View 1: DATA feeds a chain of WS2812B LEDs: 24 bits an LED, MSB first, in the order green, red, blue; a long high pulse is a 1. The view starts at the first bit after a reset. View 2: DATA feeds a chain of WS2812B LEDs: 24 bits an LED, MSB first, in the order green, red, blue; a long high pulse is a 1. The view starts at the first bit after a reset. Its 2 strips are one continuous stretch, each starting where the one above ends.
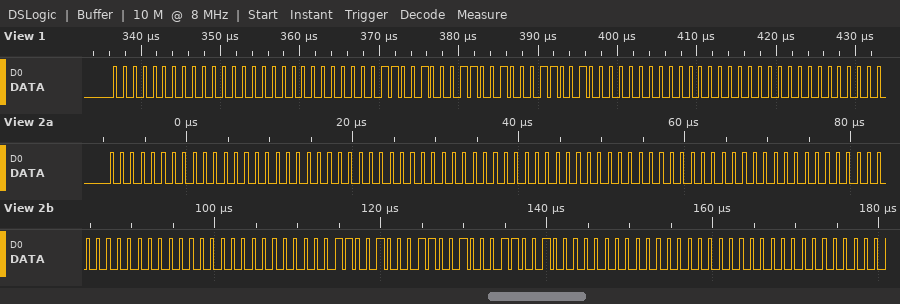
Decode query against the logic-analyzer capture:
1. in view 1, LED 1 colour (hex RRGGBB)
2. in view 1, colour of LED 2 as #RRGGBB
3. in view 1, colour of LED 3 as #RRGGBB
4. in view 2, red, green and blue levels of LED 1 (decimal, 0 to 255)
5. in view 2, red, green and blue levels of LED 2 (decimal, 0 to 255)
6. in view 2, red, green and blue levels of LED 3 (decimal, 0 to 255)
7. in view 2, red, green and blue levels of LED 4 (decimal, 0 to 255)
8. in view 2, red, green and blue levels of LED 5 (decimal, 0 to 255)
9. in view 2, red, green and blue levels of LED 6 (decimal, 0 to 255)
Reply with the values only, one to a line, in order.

#000000
#191919
#000000
0, 0, 0
0, 0, 0
0, 0, 0
0, 0, 0
25, 25, 25
0, 0, 0
